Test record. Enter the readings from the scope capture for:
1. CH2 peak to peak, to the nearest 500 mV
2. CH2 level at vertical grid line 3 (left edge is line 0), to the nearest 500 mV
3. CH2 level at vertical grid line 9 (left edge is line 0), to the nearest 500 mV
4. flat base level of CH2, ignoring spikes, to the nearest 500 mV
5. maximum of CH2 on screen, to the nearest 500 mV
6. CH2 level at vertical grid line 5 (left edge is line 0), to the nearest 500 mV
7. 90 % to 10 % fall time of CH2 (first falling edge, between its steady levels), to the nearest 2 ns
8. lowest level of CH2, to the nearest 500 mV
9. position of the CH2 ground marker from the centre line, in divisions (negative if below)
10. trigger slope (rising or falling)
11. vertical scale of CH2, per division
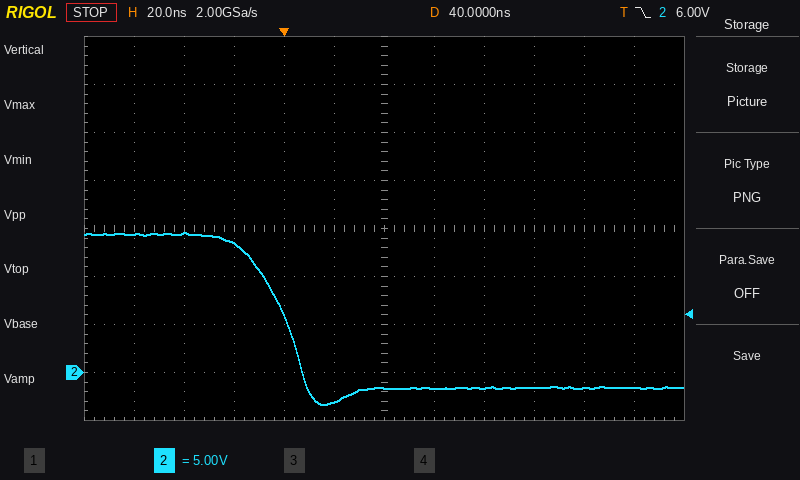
18.0 V
13.5 V
-1.5 V
-1.5 V
14.5 V
-3.0 V
24 ns
-3.5 V
-3.0 div
falling
5 V
